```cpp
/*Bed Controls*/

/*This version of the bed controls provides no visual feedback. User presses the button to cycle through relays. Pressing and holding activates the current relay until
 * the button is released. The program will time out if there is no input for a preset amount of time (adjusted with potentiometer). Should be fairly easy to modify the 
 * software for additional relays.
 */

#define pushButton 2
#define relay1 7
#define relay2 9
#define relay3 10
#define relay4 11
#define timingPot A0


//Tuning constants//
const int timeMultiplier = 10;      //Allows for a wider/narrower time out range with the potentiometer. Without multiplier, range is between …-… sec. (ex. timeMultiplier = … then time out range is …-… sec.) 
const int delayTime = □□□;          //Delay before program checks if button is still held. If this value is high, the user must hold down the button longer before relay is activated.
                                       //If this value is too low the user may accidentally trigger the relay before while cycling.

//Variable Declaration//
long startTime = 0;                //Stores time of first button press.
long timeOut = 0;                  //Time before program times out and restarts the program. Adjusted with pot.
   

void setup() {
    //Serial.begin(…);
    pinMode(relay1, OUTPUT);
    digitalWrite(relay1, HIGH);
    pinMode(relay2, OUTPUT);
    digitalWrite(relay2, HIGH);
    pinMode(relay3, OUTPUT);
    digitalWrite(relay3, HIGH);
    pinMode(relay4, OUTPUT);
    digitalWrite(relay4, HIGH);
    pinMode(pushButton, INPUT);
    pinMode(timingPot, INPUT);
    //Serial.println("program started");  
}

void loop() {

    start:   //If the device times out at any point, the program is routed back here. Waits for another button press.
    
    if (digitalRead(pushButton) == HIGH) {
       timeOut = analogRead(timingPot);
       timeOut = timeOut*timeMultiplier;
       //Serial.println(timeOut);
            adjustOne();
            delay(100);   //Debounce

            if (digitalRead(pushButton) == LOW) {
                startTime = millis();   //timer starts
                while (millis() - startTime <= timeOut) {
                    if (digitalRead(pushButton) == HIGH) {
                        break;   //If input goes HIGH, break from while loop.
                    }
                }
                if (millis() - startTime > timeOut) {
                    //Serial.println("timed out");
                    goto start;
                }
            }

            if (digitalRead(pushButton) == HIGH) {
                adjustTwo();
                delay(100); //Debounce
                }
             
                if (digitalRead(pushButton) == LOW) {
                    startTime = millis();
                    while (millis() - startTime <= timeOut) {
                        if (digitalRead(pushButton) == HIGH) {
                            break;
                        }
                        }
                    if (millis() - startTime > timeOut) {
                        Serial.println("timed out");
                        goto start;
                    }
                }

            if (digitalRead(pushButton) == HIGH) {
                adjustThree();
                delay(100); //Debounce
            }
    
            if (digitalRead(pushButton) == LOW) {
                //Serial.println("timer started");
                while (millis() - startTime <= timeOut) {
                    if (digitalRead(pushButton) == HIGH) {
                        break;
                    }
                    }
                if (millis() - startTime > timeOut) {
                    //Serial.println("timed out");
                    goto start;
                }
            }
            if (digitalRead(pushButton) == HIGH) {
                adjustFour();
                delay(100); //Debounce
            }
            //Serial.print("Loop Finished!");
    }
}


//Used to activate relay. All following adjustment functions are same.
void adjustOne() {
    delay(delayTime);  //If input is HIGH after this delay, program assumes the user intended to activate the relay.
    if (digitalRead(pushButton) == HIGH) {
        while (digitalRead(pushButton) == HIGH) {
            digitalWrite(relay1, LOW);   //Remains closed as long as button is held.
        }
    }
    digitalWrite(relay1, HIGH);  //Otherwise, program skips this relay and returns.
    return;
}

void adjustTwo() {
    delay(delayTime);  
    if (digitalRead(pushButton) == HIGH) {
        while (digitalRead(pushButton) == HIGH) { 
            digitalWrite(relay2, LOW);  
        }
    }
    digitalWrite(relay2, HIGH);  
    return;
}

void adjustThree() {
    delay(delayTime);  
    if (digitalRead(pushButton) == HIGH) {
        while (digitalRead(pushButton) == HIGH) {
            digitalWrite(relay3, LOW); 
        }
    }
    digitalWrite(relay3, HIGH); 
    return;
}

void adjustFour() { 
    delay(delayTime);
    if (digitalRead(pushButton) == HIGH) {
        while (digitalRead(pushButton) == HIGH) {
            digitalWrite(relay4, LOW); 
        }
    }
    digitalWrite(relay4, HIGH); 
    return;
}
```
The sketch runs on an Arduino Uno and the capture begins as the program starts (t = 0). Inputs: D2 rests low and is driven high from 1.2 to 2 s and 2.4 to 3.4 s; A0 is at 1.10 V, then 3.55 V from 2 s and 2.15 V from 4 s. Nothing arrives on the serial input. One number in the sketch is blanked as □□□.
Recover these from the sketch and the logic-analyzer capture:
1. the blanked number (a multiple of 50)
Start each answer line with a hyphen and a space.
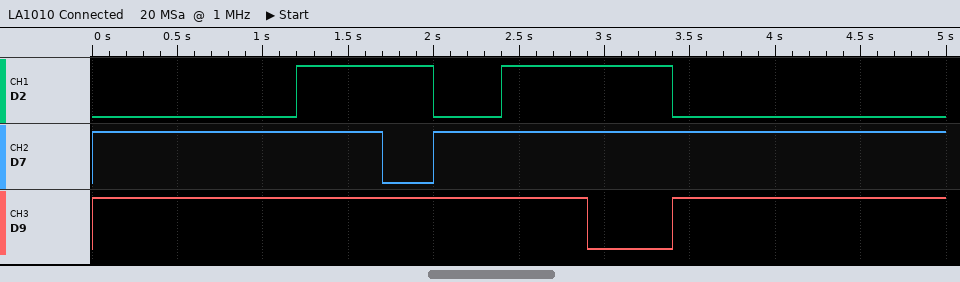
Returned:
- 500
